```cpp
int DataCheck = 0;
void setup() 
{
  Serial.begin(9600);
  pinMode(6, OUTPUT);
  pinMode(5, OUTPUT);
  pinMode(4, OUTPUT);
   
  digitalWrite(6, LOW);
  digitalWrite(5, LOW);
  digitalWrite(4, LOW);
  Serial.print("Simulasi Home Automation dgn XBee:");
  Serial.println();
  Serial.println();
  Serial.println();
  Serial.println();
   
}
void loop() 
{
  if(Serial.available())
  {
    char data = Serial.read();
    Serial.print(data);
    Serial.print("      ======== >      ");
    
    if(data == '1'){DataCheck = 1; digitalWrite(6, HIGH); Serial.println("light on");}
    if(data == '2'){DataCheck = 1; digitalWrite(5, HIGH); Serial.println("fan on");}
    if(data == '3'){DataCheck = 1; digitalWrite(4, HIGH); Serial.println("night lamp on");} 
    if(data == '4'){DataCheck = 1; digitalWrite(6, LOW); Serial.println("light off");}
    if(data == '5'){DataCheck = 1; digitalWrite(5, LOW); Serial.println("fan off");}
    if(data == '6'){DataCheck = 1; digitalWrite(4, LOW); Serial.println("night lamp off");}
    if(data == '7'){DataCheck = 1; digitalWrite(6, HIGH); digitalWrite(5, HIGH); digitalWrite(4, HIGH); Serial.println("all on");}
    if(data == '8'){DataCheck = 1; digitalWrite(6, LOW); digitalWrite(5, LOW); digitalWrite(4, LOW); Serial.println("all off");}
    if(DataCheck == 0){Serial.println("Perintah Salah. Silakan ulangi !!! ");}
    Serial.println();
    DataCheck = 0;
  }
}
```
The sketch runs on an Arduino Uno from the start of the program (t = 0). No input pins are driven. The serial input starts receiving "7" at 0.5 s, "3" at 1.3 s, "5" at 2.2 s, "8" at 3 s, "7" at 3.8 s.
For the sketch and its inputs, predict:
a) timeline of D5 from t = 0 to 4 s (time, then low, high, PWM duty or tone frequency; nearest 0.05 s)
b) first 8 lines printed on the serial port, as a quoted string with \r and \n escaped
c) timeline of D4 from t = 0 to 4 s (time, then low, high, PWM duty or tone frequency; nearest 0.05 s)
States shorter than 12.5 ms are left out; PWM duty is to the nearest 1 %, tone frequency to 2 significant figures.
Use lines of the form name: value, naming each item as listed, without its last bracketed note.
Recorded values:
timeline of D5 from t = 0 to 4 s: 0 s low; 0.5 s high; 2.2 s low; 3.8 s high
first 8 lines printed on the serial port, as a quoted string with \r and \n escaped: "Simulasi Home Automation dgn XBee:\r\n\r\n\r\n\r\n7      ======== >      all on\r\n\r\n3      ======== >      night lamp on\r\n\r\n"
timeline of D4 from t = 0 to 4 s: 0 s low; 0.5 s high; 3 s low; 3.8 s high
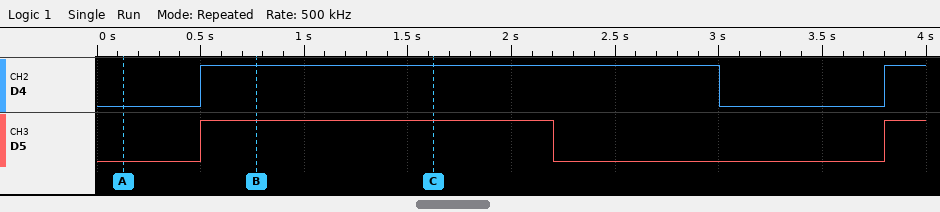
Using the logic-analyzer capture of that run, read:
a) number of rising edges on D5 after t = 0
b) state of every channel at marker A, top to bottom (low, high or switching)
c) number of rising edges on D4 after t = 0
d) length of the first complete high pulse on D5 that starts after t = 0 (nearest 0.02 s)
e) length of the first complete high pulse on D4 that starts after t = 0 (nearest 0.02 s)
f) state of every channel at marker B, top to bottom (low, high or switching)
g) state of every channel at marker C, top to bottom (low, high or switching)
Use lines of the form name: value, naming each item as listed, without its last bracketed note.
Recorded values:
number of rising edges on D5 after t = 0: 2
state of every channel at marker A, top to bottom: D4 low, D5 low
number of rising edges on D4 after t = 0: 2
length of the first complete high pulse on D5 that starts after t = 0: 1.70 s
length of the first complete high pulse on D4 that starts after t = 0: 2.50 s
state of every channel at marker B, top to bottom: D4 high, D5 high
state of every channel at marker C, top to bottom: D4 high, D5 high
